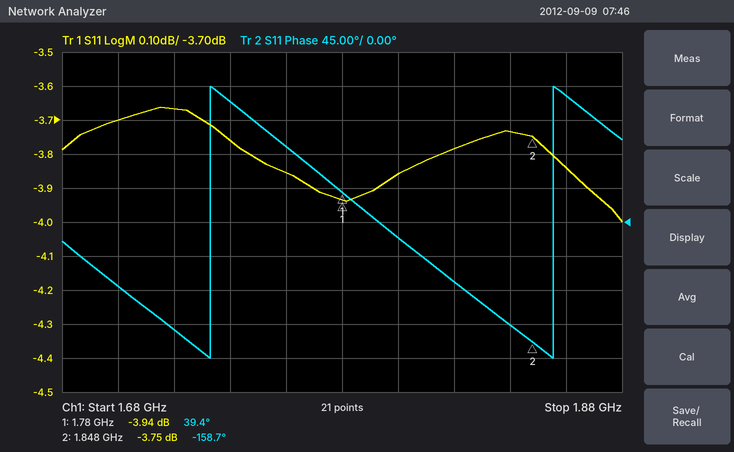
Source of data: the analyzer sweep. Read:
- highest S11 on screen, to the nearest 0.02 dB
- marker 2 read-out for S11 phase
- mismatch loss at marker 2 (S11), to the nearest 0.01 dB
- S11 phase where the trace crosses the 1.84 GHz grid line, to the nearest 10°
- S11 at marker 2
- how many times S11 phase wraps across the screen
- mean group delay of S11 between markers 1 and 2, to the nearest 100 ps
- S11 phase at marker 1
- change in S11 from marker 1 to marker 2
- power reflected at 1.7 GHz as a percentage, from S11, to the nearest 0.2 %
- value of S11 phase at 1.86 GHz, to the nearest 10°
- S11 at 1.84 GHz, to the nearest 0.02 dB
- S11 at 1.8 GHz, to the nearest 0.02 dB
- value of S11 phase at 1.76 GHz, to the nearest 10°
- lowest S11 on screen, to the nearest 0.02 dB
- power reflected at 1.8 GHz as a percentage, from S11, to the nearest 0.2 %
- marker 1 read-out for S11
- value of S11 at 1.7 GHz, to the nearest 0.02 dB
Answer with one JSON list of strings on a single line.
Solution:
["-3.66 dB", "-158.7°", "2.38 dB", "-140°", "-3.75 dB", "2", "8.1 ns", "39.4°", "0.19 dB", "42.6 %", "170°", "-3.74 dB", "-3.86 dB", "100°", "-4.00 dB", "41.2 %", "-3.94 dB", "-3.70 dB"]
